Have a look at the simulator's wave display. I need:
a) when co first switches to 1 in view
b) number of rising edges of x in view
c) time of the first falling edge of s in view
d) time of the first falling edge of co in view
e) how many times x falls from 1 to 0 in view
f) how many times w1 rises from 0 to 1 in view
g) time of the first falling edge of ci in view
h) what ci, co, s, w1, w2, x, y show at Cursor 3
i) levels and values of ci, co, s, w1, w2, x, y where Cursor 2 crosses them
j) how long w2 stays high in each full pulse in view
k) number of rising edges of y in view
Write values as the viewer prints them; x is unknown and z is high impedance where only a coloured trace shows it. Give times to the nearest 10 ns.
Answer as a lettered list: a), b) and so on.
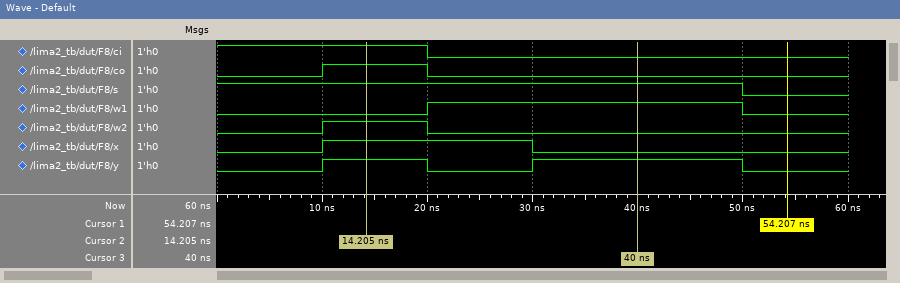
a) 10 ns
b) 1
c) 50 ns
d) 20 ns
e) 1
f) 1
g) 20 ns
h) ci=0, co=0, s=1, w1=1, w2=0, x=0, y=1
i) ci=1, co=1, s=1, w1=0, w2=1, x=1, y=1
j) 10 ns
k) 2
